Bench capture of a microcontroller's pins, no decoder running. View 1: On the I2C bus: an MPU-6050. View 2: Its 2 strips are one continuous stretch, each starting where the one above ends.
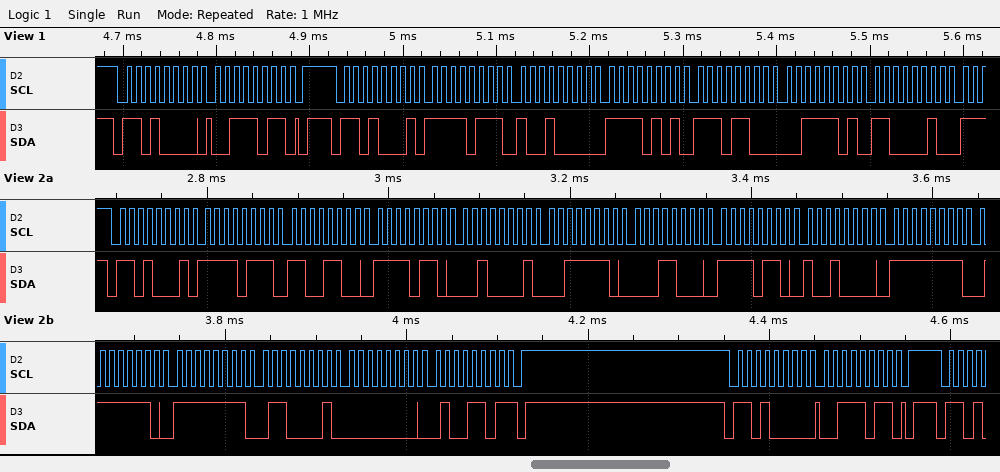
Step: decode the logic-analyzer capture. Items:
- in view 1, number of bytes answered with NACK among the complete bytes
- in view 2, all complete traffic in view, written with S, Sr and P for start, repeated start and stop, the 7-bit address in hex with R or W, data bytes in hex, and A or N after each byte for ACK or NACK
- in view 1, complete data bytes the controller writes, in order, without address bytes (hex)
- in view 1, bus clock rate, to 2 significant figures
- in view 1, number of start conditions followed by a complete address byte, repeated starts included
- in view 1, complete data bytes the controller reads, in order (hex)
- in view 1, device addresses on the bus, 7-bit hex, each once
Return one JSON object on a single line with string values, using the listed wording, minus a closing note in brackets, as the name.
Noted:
{"in view 1, number of bytes answered with NACK among the complete bytes": "0", "in view 2, all complete traffic in view, written with S, Sr and P for start, repeated start and stop, the 7-bit address in hex with R or W, data bytes in hex, and A or N after each byte for ACK or NACK": "S 68R A F7 A CC A F6 A 21 A 3E A 18 A F6 A 90 A FF A 7E A FF A 61 A 00 A 4D N P S 68W A 3B A P", "in view 1, complete data bytes the controller writes, in order, without address bytes": "3B", "in view 1, bus clock rate, to 2 significant figures": "100 kHz", "in view 1, number of start conditions followed by a complete address byte, repeated starts included": "2", "in view 1, complete data bytes the controller reads, in order": "F7 90 F5 EC 3D C2", "in view 1, device addresses on the bus, 7-bit hex, each once": "0x68"}
